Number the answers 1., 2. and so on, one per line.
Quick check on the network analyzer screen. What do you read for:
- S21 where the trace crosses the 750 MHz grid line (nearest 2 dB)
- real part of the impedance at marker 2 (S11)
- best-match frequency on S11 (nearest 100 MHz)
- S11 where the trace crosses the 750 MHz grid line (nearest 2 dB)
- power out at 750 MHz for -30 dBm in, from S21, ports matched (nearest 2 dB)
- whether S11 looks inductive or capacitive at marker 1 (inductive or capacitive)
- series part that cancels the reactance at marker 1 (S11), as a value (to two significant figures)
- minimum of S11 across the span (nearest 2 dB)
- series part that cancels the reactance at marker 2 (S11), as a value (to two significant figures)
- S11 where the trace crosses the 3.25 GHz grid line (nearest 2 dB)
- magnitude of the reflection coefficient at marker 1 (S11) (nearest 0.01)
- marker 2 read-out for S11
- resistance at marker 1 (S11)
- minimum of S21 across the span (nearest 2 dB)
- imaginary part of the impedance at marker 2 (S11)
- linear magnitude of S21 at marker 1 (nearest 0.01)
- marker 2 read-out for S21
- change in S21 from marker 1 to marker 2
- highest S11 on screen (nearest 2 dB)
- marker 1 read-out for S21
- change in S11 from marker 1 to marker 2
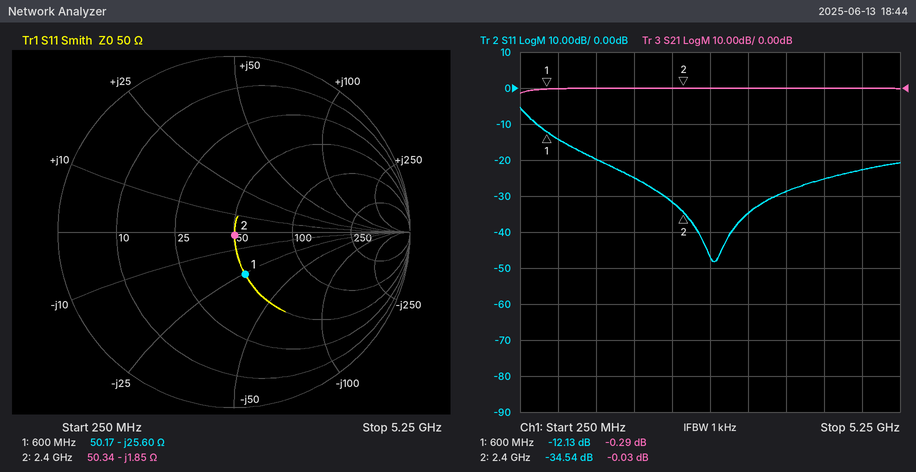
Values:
1. 0 dB
2. 50.34 Ω
3. 2.8 GHz
4. -14 dB
5. -30 dBm
6. capacitive
7. 6.8 nH
8. -48 dB
9. 120 pH
10. -34 dB
11. 0.25
12. -34.54 dB
13. 50.17 Ω
14. -2 dB
15. -1.85 Ω
16. 0.97
17. -0.03 dB
18. 0.26 dB
19. -6 dB
20. -0.29 dB
21. -22.41 dB
